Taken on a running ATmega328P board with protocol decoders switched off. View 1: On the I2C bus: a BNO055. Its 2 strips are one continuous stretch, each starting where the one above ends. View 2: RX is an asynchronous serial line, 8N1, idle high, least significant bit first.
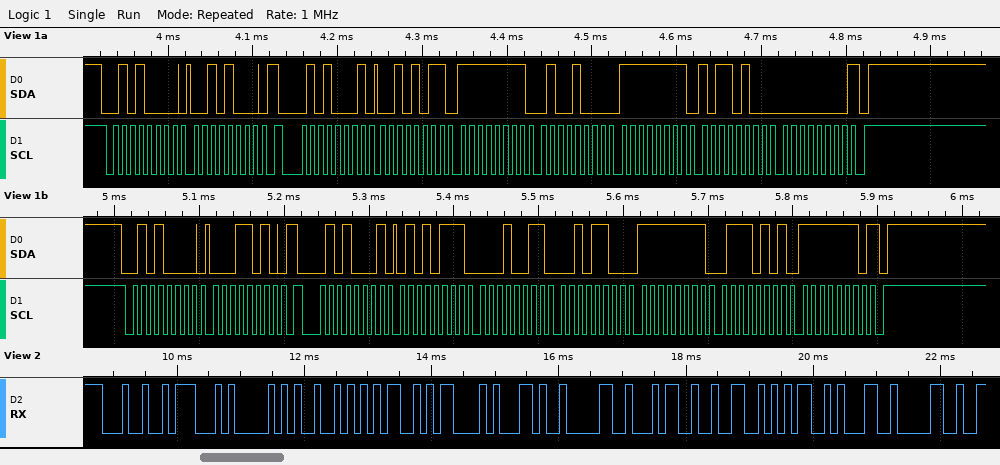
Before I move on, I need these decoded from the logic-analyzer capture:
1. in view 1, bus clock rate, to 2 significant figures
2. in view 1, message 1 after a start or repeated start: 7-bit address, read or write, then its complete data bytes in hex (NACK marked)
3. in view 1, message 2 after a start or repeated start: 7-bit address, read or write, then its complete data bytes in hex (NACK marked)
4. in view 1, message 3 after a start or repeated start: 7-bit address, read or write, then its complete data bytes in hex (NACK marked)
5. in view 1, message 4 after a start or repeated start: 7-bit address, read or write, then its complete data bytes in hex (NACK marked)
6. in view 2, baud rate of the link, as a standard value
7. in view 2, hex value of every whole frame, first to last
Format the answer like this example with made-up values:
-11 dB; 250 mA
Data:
100 kHz; 0x28 write: 28; 0x28 read: 2B FF 48 FF B4 00 NACK; 0x28 write: 1A; 0x28 read: 57 13 2C FF 75 FE NACK; 9600 baud; 24 47 50 52 4D 43 2C 30 34 32 35 31 30
